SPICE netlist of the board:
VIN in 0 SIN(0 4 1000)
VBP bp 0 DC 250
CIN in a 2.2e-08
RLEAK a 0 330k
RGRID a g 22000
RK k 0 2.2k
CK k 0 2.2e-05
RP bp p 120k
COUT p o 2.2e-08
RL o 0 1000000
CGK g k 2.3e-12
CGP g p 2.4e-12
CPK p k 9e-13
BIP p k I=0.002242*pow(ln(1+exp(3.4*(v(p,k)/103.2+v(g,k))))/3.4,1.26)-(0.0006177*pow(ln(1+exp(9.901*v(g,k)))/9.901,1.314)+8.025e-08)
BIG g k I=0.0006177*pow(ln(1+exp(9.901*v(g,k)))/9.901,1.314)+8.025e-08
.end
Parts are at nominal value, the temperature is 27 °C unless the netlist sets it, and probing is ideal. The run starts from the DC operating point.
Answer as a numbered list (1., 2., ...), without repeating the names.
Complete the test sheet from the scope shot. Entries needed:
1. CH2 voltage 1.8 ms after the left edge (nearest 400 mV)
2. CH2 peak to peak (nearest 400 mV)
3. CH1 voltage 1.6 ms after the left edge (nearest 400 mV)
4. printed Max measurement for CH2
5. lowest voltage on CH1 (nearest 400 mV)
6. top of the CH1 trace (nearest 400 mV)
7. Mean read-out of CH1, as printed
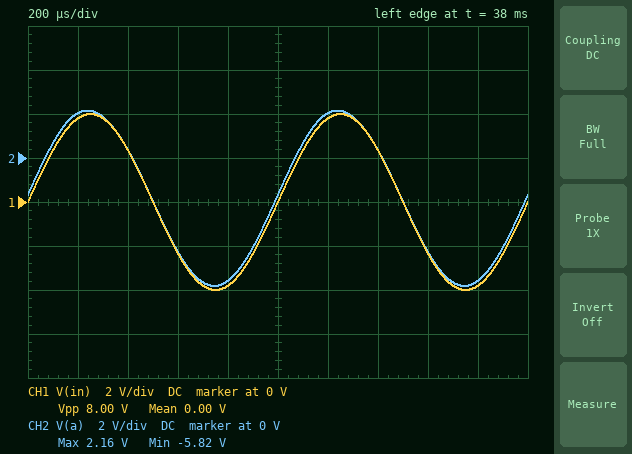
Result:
1. -5.6 V
2. 8.0 V
3. -2.4 V
4. 2.16 V
5. -4.0 V
6. 4.0 V
7. 0.00 V
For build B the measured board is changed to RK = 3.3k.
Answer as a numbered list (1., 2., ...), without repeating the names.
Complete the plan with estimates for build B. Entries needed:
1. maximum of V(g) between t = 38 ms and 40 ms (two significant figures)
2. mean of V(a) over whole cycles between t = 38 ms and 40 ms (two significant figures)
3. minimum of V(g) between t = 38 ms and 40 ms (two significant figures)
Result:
1. 1.7 V
2. -1.5 V
3. -5.5 V
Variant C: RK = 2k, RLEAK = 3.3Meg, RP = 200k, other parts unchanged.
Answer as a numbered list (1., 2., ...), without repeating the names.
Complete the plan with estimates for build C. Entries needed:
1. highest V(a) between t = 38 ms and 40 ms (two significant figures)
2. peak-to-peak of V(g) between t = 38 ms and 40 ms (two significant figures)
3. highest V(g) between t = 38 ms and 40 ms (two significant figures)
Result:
1. 940 mV
2. 7.8 V
3. 710 mV
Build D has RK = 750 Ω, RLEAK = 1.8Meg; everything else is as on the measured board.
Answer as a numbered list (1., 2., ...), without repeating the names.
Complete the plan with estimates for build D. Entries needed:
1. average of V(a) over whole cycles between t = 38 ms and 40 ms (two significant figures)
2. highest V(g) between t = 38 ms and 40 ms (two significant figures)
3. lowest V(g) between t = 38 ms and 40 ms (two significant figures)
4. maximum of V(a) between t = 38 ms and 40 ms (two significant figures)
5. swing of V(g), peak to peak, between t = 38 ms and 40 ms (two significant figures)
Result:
1. -3.3 V
2. 360 mV
3. -7.3 V
4. 720 mV
5. 7.6 V
